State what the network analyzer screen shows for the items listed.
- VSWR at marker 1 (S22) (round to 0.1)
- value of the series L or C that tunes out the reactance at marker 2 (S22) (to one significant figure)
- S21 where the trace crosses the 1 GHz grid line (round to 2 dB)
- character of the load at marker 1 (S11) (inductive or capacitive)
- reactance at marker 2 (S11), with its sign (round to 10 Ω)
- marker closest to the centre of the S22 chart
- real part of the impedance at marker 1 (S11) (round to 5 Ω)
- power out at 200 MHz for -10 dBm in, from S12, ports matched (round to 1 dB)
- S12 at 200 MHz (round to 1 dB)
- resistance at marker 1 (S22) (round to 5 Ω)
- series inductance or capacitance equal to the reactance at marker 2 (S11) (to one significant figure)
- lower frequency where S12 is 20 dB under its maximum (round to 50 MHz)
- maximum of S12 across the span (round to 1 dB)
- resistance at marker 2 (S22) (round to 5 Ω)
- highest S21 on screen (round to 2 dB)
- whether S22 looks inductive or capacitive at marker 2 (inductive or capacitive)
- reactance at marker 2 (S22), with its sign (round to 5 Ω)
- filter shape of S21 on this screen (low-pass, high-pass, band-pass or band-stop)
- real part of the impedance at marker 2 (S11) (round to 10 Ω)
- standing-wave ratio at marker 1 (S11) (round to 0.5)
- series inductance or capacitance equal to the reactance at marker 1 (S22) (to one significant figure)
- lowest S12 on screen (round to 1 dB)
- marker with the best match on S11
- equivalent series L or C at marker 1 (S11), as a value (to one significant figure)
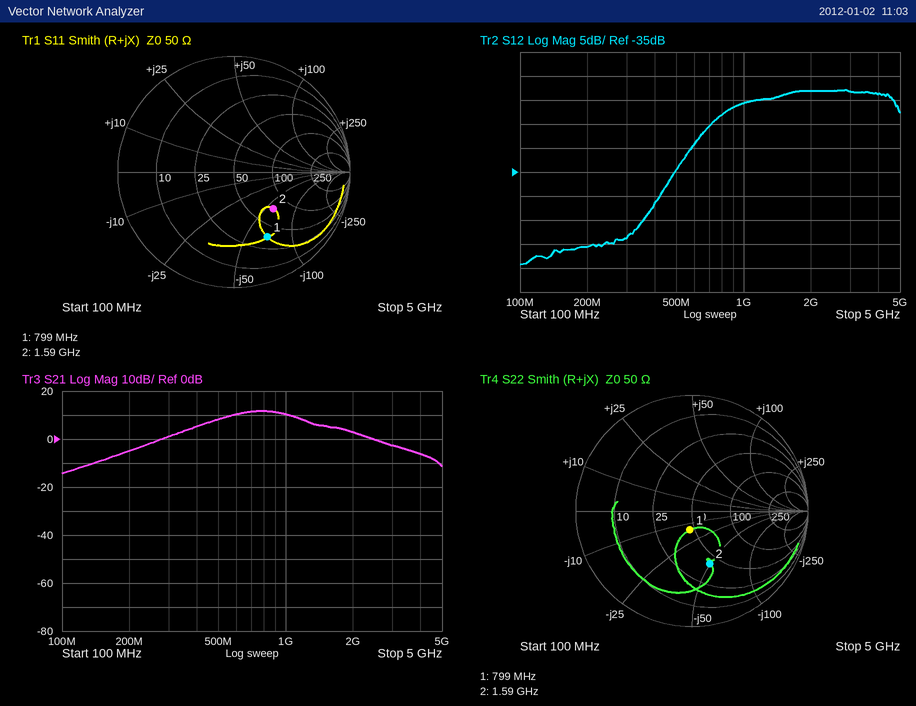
1.4
5 nH
10 dB
capacitive
-60 Ω
marker 1
35 Ω
-61 dBm
-51 dB
45 Ω
2 pF
450 MHz
-18 dB
40 Ω
12 dB
capacitive
-50 Ω
band-pass
70 Ω
4.5
10 pF
-54 dB
marker 2
3 pF
